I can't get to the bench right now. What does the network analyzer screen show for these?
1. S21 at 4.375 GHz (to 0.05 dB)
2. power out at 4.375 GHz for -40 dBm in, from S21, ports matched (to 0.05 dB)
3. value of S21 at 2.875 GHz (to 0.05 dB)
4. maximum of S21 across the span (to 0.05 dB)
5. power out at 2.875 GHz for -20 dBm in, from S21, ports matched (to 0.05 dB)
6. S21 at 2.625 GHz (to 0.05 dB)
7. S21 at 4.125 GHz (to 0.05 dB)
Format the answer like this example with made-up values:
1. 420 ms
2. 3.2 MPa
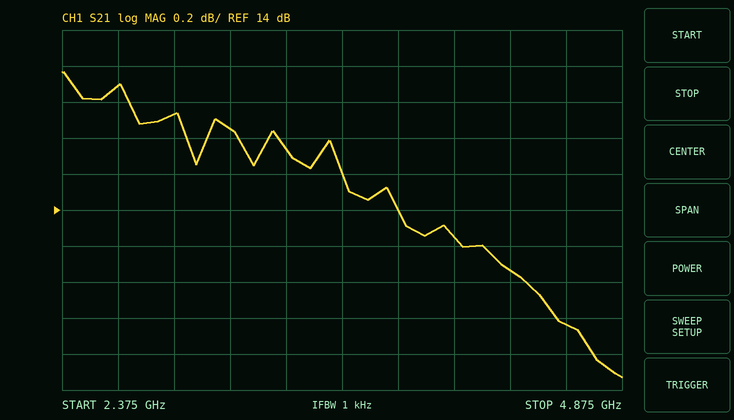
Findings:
1. 13.65 dB
2. -26.35 dBm
3. 14.55 dB
4. 14.75 dB
5. -5.45 dBm
6. 14.70 dB
7. 13.85 dB
